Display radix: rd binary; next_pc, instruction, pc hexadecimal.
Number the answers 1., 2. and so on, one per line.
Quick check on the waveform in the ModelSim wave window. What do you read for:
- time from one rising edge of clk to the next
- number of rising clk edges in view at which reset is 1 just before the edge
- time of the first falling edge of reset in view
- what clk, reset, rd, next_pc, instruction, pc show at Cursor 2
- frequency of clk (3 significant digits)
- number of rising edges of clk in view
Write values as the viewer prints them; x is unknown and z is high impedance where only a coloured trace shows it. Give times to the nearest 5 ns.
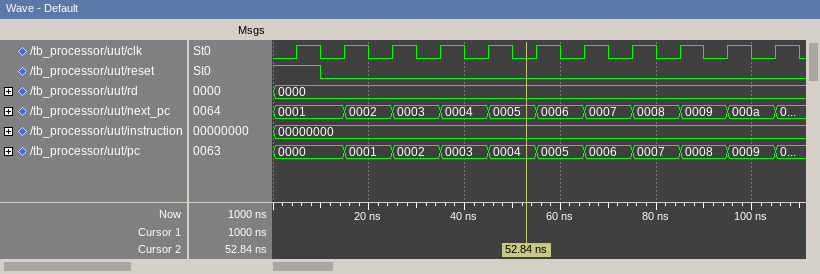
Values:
1. 10 ns
2. 1
3. 10 ns
4. clk=0, reset=0, rd=0000, next_pc=0005, instruction=00000000, pc=0004
5. 100 MHz
6. 11
